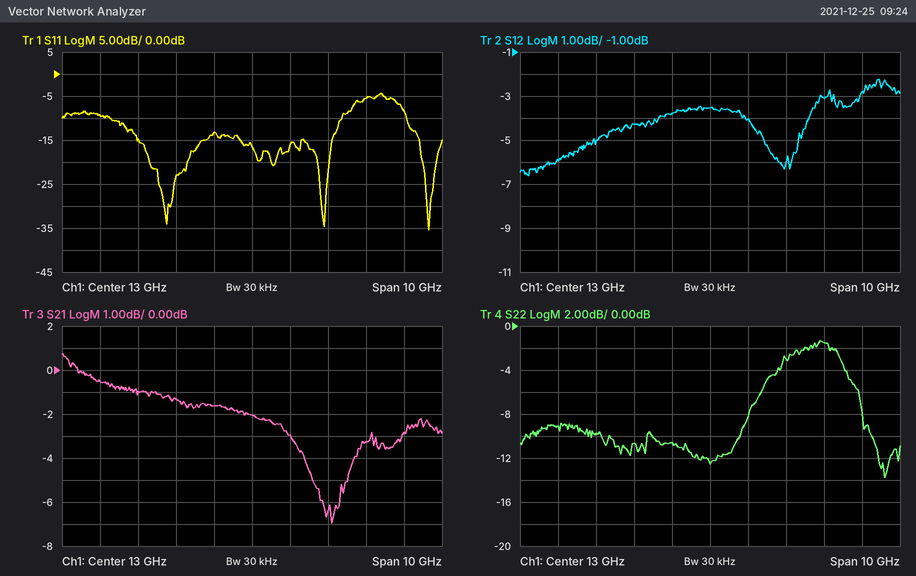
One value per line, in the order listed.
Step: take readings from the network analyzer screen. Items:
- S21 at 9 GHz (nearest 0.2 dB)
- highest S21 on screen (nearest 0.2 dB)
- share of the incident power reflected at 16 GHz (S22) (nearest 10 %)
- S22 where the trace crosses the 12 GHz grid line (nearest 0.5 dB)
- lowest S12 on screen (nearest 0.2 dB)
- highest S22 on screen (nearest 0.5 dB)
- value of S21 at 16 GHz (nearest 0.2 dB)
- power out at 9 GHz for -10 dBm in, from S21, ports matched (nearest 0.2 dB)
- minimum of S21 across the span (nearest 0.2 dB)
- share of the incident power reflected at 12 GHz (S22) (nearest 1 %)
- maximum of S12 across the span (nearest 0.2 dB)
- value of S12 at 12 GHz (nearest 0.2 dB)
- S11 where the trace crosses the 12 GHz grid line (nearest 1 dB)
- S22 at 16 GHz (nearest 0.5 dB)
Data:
-0.6 dB
0.8 dB
70 %
-10.5 dB
-6.6 dB
-1.5 dB
-3.2 dB
-10.6 dBm
-7.0 dB
9 %
-2.2 dB
-3.8 dB
-13 dB
-1.5 dB
